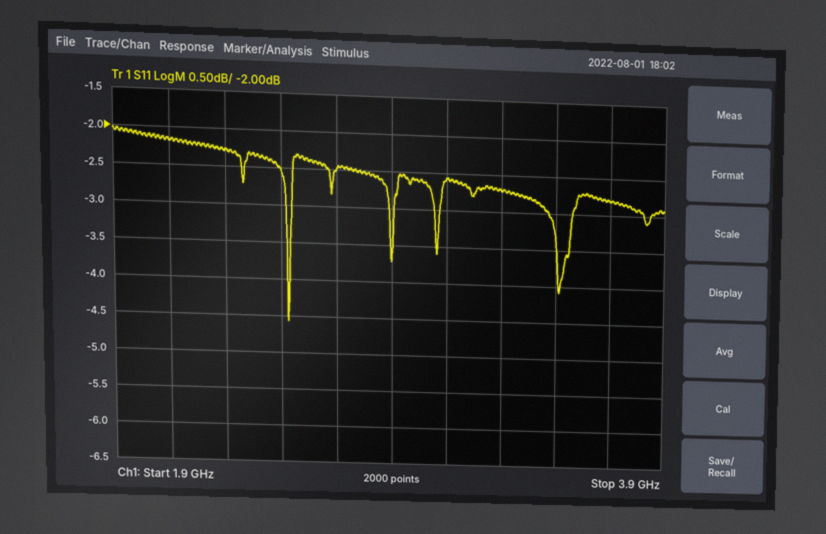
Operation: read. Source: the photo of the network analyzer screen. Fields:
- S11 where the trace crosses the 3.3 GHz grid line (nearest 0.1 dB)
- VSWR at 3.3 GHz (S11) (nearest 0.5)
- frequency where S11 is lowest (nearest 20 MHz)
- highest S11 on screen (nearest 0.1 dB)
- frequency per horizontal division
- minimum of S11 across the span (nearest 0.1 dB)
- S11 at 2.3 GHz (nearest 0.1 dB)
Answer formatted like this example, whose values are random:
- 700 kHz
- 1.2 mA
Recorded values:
- -2.7 dB
- 6.5
- 2.52 GHz
- -2.0 dB
- 200 MHz
- -4.6 dB
- -2.3 dB
